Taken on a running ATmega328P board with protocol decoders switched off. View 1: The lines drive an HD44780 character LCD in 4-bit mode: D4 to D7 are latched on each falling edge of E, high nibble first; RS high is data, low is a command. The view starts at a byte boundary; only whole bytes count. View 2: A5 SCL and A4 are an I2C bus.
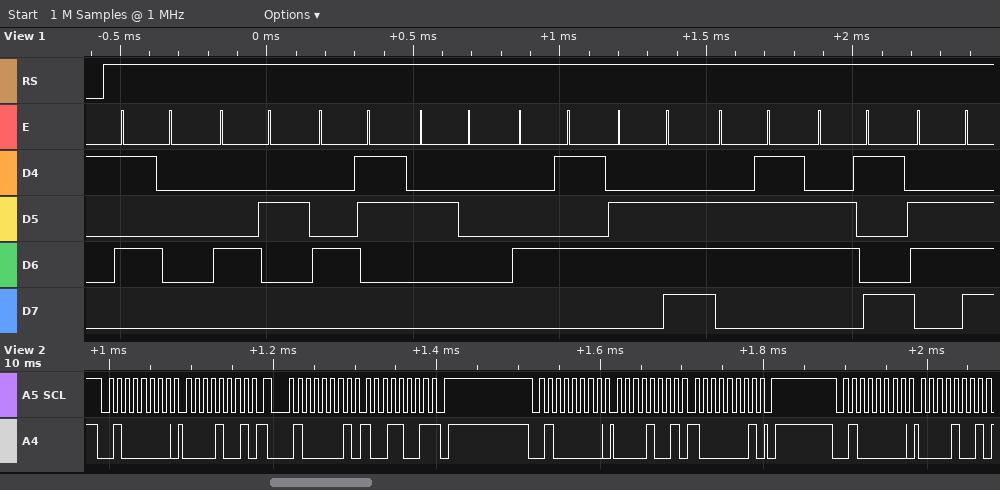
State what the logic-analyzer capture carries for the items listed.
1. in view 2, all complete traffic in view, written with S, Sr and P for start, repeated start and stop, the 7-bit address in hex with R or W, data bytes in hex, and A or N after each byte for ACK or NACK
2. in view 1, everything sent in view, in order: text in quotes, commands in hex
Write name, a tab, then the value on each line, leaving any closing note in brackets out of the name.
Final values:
in view 2, all complete traffic in view, written with S, Sr and P for start, repeated start and stop, the 7-bit address in hex with R or W, data bytes in hex, and A or N after each byte for ACK or NACK	S 20W A 09 A Sr 20R A 99 N P S 20W A 09 A 81 A P S 20W A 09 A
in view 1, everything sent in view, in order: text in quotes, commands in hex	"PBC Engin"
